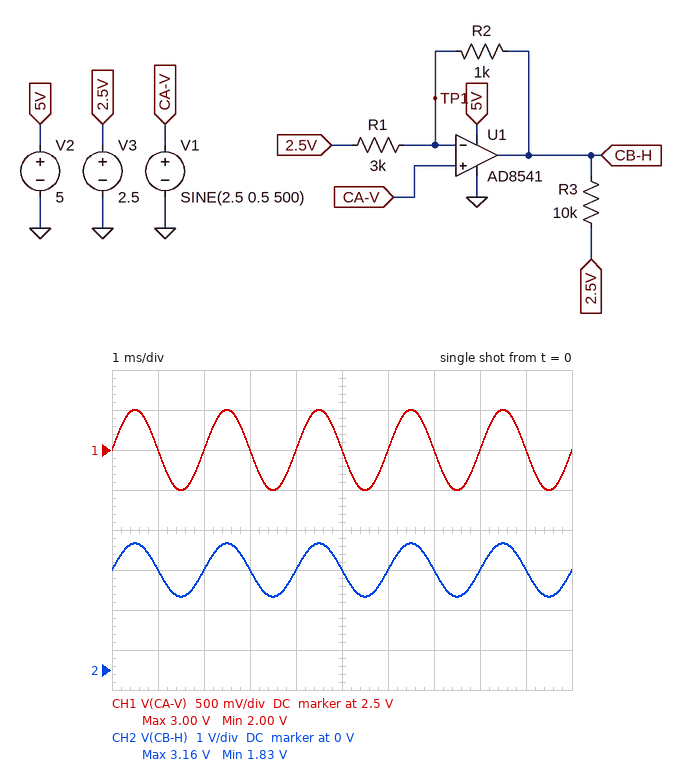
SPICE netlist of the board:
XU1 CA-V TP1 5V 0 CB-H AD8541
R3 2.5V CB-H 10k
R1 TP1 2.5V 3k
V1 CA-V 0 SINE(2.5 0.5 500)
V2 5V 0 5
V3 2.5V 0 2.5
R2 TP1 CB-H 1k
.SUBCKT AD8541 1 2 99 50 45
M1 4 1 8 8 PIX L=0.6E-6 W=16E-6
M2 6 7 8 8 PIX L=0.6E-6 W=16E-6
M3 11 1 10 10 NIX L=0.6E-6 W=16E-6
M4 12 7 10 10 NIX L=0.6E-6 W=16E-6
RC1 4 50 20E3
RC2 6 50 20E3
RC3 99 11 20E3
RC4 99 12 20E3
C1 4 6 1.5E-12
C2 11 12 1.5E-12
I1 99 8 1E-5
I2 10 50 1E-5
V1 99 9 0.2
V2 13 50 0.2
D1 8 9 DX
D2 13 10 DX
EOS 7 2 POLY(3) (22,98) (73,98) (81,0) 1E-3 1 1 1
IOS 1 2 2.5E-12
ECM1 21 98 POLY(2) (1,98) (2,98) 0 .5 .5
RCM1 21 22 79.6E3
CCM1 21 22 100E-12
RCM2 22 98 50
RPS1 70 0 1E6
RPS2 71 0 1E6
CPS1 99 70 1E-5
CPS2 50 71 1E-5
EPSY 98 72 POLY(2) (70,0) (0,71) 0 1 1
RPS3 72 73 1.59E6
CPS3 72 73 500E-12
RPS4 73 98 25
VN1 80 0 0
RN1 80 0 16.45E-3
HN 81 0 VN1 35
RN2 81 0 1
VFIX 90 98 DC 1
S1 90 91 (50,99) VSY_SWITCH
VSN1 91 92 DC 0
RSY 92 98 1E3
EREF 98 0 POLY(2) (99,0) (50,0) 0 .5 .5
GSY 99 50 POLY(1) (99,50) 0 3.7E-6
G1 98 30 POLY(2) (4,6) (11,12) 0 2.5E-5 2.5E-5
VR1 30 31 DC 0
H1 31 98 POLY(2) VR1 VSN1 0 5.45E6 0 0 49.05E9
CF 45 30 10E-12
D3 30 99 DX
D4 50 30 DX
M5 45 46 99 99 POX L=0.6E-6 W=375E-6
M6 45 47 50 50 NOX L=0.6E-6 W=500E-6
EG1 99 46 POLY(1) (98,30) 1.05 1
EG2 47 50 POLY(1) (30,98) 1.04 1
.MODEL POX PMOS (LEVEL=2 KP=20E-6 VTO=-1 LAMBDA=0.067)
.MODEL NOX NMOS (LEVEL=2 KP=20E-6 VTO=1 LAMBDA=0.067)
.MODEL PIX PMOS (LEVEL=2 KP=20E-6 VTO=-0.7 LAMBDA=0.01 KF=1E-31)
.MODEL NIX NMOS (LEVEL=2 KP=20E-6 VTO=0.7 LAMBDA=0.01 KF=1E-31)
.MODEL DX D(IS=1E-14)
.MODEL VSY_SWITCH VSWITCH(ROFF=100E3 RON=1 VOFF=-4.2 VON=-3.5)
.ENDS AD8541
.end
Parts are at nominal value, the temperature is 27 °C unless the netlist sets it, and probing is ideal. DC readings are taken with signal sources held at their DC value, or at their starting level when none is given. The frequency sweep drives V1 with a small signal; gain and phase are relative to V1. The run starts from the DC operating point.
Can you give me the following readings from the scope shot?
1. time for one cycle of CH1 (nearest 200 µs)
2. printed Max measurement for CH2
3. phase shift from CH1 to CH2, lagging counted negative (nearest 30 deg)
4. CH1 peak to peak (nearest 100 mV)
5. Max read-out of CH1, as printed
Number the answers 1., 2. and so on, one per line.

1. 2.0 ms
2. 3.16 V
3. 0 deg
4. 1.0 V
5. 3.00 V
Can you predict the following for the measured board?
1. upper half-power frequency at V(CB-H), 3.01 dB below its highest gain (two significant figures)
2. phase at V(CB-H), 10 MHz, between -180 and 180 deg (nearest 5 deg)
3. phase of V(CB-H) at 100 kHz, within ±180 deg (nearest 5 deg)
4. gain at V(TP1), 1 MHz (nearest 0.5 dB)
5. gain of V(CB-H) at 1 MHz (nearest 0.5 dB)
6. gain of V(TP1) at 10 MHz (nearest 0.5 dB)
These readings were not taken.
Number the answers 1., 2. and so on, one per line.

1. 970 kHz
2. 165 deg
3. -10 deg
4. -3.0 dB
5. -0.5 dB
6. -34.0 dB
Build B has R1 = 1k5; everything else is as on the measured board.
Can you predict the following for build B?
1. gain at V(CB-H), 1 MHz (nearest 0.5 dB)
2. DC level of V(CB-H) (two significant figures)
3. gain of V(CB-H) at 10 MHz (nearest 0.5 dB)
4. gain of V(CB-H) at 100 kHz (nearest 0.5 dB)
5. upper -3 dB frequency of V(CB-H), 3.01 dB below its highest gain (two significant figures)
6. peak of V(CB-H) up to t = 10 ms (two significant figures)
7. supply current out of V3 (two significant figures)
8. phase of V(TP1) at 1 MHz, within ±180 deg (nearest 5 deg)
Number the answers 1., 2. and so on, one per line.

1. -1.0 dB
2. 2.5 V
3. -32.5 dB
4. 4.5 dB
5. 670 kHz
6. 3.3 V
7. 830 nA
8. -85 deg
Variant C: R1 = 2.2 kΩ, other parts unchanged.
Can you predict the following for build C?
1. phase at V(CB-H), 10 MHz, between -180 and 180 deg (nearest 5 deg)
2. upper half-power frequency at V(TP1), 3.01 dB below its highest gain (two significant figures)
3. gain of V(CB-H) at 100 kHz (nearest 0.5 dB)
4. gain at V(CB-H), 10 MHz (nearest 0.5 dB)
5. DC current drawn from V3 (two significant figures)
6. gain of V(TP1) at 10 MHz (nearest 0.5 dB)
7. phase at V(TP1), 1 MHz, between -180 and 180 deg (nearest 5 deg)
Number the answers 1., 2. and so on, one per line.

1. 165 deg
2. 840 kHz
3. 3.0 dB
4. -32.0 dB
5. 600 nA
6. -35.0 dB
7. -80 deg
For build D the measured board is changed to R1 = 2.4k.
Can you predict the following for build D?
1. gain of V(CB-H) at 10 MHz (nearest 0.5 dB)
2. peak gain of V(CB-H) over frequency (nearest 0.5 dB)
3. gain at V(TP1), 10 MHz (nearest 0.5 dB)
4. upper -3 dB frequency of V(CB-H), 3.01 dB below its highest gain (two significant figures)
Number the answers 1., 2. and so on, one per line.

1. -32.0 dB
2. 3.0 dB
3. -35.0 dB
4. 880 kHz
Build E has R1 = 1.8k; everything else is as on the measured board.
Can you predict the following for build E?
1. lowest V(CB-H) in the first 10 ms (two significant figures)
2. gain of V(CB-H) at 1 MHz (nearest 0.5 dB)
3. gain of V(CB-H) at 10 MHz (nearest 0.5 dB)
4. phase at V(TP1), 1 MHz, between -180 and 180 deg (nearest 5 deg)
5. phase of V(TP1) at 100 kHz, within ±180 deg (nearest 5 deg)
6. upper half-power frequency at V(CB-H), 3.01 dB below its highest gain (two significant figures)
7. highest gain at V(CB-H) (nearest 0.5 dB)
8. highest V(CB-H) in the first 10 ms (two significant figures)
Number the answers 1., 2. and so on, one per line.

1. 1.7 V
2. -1.0 dB
3. -32.0 dB
4. -80 deg
5. -10 deg
6. 750 kHz
7. 4.0 dB
8. 3.3 V
